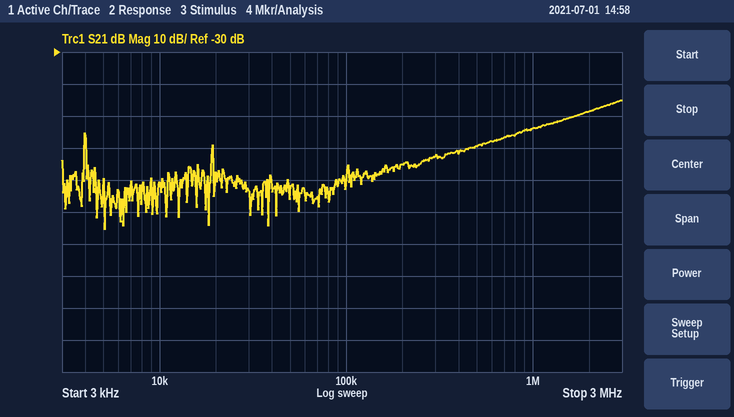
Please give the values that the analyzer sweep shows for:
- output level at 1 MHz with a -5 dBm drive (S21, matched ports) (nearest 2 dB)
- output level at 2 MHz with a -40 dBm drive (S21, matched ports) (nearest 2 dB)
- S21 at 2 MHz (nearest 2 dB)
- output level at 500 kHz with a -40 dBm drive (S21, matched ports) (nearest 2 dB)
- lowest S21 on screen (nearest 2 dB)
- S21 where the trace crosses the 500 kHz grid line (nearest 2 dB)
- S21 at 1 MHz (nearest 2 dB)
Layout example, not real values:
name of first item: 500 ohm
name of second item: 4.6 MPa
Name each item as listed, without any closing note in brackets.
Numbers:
output level at 1 MHz with a -5 dBm drive (S21, matched ports): -58 dBm
output level at 2 MHz with a -40 dBm drive (S21, matched ports): -88 dBm
S21 at 2 MHz: -48 dB
output level at 500 kHz with a -40 dBm drive (S21, matched ports): -100 dBm
lowest S21 on screen: -86 dB
S21 where the trace crosses the 500 kHz grid line: -60 dB
S21 at 1 MHz: -54 dB
